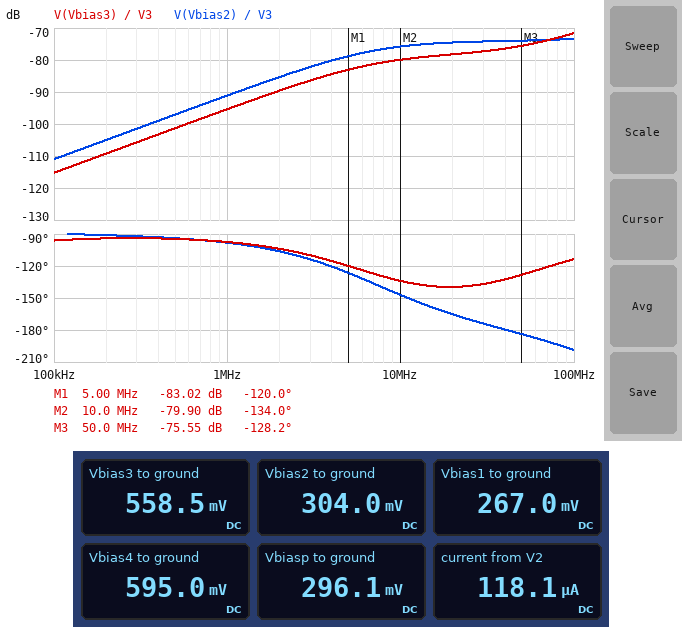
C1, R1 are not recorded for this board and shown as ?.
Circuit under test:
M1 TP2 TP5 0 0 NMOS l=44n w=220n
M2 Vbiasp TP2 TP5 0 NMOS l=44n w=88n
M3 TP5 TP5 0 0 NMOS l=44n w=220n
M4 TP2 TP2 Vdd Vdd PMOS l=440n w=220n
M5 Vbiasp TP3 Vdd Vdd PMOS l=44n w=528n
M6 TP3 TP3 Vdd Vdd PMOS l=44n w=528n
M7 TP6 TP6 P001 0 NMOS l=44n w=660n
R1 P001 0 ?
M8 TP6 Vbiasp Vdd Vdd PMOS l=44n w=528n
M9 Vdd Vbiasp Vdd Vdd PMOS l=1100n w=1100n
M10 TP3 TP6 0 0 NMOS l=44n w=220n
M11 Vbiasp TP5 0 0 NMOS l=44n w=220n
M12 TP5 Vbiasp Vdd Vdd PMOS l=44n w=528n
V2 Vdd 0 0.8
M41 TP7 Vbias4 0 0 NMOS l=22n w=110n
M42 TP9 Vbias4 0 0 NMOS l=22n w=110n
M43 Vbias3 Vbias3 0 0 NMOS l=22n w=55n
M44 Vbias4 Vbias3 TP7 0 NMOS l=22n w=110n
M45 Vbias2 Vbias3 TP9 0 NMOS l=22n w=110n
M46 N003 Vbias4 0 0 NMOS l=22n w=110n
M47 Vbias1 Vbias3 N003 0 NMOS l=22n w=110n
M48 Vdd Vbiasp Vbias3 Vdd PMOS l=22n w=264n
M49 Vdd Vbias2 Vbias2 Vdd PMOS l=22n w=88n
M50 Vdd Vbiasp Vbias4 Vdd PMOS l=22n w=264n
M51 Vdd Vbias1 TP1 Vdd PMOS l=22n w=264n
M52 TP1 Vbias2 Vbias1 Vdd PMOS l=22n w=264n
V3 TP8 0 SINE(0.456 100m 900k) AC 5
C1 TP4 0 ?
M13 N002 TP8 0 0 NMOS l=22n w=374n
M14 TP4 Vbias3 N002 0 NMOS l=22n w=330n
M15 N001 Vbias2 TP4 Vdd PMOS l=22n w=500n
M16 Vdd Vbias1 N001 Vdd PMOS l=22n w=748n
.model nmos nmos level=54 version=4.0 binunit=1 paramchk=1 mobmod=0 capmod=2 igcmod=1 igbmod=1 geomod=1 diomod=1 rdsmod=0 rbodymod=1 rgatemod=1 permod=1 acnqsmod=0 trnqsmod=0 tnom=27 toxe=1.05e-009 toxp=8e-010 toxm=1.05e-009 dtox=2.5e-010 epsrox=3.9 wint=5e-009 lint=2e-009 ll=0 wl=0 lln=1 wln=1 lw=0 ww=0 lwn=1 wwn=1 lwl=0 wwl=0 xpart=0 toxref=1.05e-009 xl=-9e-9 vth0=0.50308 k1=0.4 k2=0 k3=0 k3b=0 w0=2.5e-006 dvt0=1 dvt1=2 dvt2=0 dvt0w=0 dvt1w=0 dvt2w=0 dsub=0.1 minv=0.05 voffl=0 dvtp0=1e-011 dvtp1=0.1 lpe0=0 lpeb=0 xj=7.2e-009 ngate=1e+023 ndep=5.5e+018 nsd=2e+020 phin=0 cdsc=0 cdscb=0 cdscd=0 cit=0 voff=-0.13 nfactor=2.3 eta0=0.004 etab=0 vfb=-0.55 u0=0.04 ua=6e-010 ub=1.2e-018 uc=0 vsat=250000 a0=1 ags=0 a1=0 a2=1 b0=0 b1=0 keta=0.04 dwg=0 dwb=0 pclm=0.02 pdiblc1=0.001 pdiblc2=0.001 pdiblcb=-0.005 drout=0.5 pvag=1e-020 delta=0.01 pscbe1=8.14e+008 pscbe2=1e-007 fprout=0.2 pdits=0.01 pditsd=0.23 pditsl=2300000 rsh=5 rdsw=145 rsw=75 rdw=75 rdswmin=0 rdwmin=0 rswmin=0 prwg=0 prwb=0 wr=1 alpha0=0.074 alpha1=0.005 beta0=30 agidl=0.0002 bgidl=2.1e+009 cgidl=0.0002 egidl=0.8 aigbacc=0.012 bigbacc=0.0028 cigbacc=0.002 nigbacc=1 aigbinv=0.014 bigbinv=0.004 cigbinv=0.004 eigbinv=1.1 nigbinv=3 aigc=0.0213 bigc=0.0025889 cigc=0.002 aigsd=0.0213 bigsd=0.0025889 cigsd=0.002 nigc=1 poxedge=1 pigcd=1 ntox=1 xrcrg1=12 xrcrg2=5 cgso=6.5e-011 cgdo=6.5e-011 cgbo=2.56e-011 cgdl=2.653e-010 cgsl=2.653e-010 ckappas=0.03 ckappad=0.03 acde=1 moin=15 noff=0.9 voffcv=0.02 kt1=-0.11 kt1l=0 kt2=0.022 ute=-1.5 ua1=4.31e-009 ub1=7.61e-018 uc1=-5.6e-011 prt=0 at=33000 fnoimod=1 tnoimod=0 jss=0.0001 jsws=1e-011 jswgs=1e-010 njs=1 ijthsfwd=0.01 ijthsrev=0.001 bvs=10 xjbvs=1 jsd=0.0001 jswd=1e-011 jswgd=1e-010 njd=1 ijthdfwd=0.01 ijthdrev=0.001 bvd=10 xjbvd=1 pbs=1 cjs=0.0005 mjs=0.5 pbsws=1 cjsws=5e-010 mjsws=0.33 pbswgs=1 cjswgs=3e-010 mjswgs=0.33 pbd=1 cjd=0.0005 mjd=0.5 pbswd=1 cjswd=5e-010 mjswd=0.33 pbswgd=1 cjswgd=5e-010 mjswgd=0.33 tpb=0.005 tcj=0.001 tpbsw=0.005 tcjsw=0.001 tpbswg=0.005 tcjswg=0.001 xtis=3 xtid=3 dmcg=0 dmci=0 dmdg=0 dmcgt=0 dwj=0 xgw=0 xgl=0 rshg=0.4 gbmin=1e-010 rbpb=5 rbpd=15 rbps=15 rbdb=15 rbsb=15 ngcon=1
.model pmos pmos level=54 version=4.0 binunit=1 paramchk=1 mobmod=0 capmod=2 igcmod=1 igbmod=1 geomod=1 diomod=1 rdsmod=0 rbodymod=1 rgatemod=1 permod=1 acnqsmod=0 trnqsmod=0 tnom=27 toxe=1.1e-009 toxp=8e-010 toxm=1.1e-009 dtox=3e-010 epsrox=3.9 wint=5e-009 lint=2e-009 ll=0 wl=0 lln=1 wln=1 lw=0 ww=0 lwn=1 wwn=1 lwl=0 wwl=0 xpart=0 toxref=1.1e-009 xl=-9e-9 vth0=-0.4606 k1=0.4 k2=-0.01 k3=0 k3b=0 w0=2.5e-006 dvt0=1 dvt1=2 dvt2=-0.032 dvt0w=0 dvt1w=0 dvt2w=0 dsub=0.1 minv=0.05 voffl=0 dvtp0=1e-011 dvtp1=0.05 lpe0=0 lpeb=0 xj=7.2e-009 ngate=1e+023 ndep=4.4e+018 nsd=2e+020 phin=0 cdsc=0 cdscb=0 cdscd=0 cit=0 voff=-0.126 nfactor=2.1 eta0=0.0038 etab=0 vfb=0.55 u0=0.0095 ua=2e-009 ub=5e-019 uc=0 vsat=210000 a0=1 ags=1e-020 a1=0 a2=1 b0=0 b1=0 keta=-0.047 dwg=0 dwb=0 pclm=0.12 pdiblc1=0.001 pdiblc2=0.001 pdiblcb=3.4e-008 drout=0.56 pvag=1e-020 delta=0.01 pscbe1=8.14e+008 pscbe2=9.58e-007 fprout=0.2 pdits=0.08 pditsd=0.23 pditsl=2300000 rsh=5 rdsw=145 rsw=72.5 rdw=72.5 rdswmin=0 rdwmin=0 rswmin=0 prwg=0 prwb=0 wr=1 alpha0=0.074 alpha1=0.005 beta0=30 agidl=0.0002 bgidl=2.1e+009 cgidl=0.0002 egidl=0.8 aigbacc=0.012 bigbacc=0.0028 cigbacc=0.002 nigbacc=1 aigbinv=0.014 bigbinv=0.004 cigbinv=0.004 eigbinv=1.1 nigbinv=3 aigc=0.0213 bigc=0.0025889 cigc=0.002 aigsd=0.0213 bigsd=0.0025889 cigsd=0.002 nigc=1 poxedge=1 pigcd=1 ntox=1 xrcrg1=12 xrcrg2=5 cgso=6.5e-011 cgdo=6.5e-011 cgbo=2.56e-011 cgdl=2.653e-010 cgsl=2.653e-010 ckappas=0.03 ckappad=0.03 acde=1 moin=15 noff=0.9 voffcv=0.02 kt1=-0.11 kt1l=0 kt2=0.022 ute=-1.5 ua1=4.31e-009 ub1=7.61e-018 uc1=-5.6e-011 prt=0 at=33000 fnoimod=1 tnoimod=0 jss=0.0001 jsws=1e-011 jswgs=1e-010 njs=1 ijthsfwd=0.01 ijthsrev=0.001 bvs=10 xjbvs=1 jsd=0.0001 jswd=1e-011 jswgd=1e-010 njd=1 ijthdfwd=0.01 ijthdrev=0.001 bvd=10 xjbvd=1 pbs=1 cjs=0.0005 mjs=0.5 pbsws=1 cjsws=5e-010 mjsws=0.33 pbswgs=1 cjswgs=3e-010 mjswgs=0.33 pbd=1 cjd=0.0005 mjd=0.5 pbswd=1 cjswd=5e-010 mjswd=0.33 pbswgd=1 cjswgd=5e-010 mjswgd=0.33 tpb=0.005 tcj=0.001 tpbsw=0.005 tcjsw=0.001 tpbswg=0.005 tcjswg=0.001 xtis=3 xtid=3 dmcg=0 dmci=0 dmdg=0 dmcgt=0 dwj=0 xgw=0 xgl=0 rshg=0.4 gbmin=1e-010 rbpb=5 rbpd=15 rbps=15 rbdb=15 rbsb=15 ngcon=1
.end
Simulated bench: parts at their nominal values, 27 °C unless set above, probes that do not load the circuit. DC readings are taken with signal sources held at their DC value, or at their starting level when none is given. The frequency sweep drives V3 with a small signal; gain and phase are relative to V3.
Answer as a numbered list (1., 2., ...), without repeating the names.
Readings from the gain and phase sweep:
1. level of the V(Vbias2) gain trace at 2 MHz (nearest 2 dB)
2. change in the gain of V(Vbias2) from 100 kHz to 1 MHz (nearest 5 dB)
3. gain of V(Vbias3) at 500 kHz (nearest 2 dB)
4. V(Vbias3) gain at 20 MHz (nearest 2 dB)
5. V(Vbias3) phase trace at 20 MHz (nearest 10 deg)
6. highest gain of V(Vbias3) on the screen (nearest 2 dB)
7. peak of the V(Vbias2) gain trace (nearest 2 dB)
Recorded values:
1. -86 dB
2. 20 dB
3. -102 dB
4. -78 dB
5. -140 deg
6. -72 dB
7. -74 dB
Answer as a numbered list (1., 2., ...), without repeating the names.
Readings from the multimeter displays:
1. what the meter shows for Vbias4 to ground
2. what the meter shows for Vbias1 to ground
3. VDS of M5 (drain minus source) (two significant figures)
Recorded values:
1. 595.0 mV
2. 267.0 mV
3. -500 mV
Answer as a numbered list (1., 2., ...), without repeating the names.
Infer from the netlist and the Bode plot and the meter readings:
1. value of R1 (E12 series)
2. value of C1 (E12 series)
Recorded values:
1. 10 kΩ
2. 1.5 pF
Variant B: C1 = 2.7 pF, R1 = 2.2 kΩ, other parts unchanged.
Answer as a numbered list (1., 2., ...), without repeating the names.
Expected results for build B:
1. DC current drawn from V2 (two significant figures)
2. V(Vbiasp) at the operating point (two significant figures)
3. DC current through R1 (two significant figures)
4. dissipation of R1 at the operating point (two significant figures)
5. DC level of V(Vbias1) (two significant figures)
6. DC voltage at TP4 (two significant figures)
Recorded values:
1. 280 µA
2. 130 mV
3. 29 µA
4. 1.8 µW
5. 210 mV
6. 640 mV
